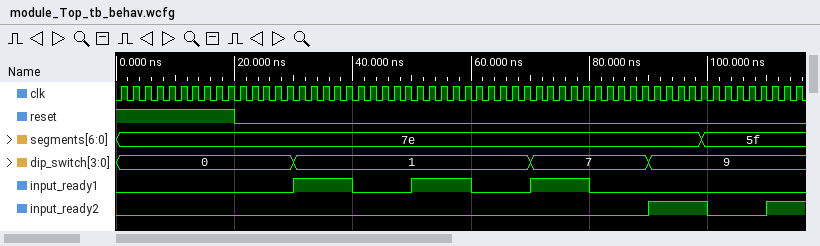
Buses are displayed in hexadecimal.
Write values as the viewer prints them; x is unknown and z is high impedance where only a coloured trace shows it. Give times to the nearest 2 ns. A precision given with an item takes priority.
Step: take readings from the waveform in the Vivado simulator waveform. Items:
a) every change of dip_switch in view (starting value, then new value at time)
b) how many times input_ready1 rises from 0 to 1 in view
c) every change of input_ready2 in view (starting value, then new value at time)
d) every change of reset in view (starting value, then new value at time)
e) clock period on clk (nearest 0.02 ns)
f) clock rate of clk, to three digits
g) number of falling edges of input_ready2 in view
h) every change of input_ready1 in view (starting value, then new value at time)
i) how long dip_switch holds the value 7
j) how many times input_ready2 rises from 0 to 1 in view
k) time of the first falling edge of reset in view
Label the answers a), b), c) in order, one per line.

a) 0, 1 at 30 ns, 7 at 70 ns, 9 at 90 ns
b) 3
c) 0, 1 at 90 ns, 0 at 100 ns, 1 at 110 ns
d) 1, 0 at 20 ns
e) 2 ns
f) 500 MHz
g) 1
h) 0, 1 at 30 ns, 0 at 40 ns, 1 at 50 ns, 0 at 60 ns, 1 at 70 ns, 0 at 80 ns
i) 20 ns
j) 2
k) 20 ns
